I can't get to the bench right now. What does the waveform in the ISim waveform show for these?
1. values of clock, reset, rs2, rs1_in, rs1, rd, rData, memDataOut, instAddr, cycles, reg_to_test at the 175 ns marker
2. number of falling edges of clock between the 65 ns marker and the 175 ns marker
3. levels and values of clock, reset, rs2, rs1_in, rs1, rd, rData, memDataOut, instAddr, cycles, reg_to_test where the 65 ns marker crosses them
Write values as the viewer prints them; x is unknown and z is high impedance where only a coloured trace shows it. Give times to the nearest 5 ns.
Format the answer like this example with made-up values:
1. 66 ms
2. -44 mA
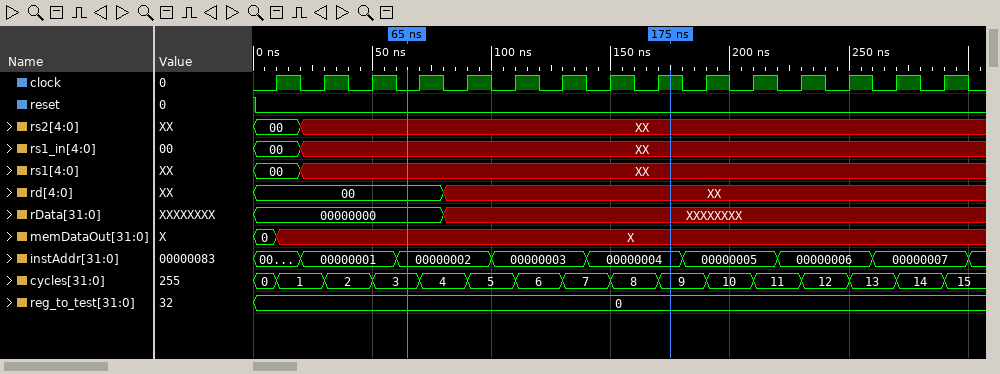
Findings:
1. clock=1, reset=0, rs2=XX, rs1_in=XX, rs1=XX, rd=XX, rData=XXXXXXXX, memDataOut=X, instAddr=00000004, cycles=9, reg_to_test=0
2. 5
3. clock=0, reset=0, rs2=XX, rs1_in=XX, rs1=XX, rd=00, rData=00000000, memDataOut=X, instAddr=00000002, cycles=3, reg_to_test=0
